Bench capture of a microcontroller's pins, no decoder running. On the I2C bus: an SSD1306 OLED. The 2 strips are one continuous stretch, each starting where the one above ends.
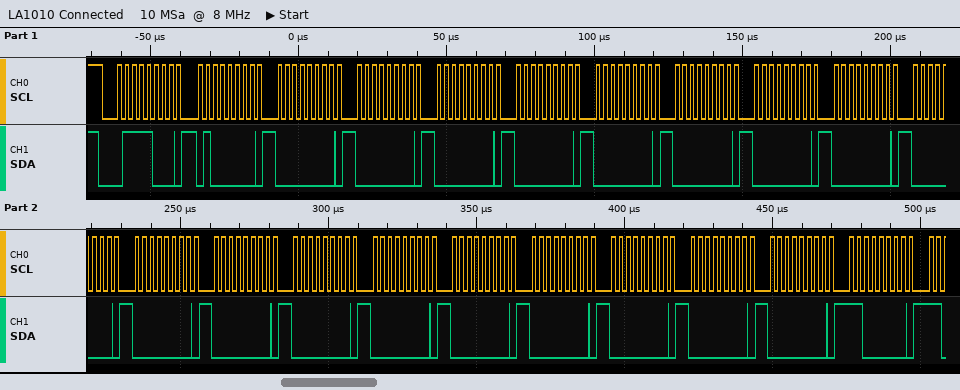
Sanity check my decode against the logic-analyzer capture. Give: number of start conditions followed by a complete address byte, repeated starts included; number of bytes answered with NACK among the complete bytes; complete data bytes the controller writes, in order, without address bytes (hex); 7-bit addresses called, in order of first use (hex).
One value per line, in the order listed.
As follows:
1
0
40 00 00 00 00 00 00 00 00 00 00 00 00 00 00 00 00 00 00 C0
0x3C
